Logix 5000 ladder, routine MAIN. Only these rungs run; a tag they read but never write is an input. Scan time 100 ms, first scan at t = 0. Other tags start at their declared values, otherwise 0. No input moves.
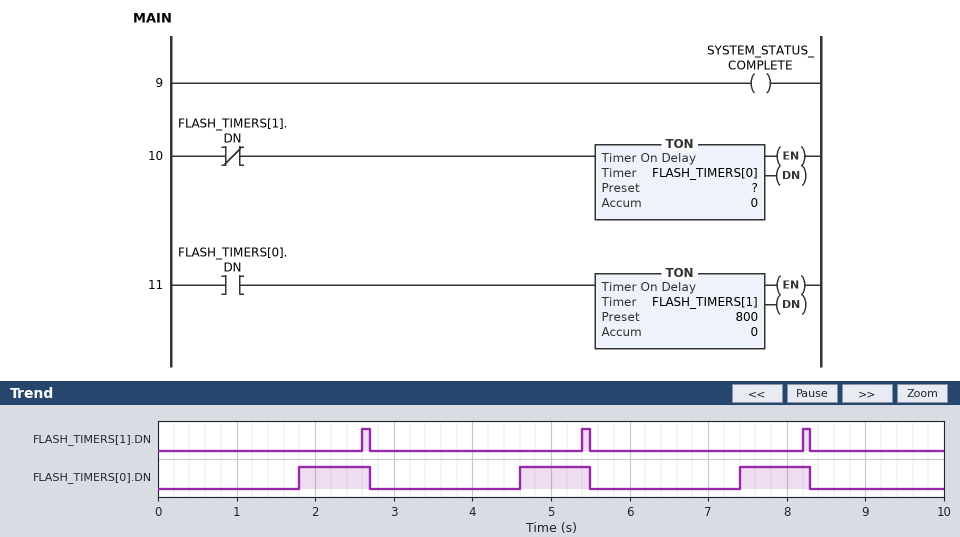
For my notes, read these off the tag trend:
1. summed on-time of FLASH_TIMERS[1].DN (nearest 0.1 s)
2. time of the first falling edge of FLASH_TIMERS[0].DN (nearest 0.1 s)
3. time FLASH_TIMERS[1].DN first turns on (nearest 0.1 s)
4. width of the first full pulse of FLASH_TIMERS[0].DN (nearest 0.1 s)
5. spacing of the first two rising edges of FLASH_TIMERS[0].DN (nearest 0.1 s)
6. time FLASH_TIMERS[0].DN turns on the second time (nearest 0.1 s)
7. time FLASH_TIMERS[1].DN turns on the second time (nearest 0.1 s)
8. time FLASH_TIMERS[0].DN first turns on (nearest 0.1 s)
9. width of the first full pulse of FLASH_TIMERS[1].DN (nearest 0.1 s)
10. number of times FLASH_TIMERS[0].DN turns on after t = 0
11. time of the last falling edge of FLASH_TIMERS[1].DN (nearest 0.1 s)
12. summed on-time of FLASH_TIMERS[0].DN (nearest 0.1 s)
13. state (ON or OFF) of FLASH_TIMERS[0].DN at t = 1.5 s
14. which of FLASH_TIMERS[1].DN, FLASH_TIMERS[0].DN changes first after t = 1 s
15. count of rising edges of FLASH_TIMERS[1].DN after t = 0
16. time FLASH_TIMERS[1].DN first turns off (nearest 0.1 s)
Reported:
0.3 s
2.7 s
2.6 s
0.9 s
2.8 s
4.6 s
5.4 s
1.8 s
0.1 s
3
8.3 s
2.7 s
OFF
FLASH_TIMERS[0].DN
3
2.7 s
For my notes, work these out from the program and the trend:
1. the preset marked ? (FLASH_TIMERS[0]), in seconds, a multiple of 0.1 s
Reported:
1.8 s
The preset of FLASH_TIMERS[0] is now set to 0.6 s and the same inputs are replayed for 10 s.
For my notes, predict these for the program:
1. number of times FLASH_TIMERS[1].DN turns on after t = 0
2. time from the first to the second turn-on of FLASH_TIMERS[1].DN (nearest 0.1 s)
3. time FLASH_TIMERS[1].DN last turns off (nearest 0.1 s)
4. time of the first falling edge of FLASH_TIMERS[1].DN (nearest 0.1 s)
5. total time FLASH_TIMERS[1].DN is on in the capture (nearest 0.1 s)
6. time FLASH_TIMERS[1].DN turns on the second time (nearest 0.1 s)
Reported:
6
1.6 s
9.5 s
1.5 s
0.6 s
3.0 s
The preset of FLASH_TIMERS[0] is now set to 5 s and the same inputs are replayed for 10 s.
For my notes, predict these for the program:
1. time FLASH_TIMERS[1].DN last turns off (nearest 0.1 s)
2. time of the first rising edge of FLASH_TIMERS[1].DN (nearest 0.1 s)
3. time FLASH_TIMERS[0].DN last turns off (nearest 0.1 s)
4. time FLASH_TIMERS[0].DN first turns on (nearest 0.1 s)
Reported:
5.9 s
5.8 s
5.9 s
5.0 s
